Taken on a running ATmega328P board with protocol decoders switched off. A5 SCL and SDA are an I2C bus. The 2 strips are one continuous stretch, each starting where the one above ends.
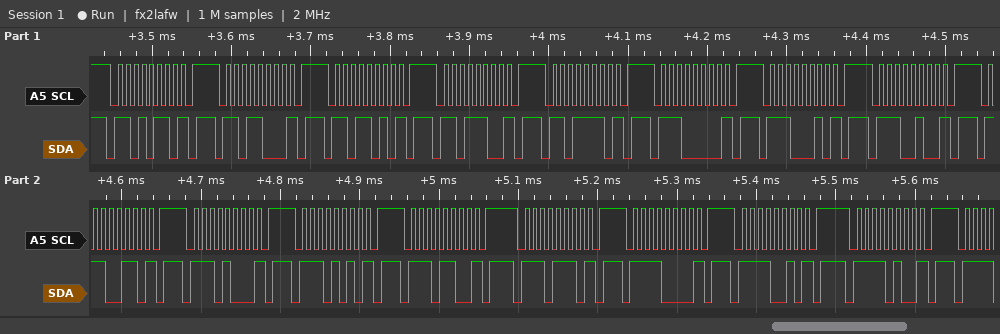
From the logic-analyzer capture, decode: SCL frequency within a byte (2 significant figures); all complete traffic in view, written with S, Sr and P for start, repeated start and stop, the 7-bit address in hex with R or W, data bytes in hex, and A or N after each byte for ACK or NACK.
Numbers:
100 kHz
S 6BW N P S 6CW N P S 6DW N P S 6EW N P S 6FW N P S 70W N P S 71W N P S 72W N P S 73W N P S 74W N P S 75W N P S 76W N P S 77W N P S 78W N P S 79W N P S 7AW N P
